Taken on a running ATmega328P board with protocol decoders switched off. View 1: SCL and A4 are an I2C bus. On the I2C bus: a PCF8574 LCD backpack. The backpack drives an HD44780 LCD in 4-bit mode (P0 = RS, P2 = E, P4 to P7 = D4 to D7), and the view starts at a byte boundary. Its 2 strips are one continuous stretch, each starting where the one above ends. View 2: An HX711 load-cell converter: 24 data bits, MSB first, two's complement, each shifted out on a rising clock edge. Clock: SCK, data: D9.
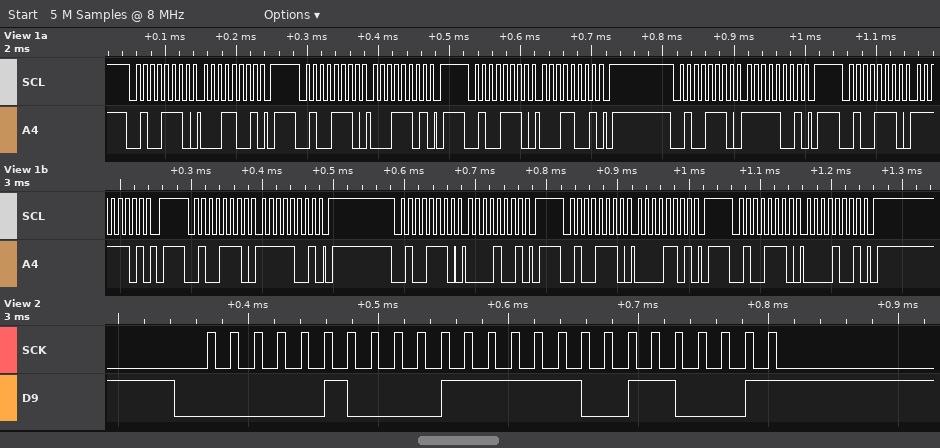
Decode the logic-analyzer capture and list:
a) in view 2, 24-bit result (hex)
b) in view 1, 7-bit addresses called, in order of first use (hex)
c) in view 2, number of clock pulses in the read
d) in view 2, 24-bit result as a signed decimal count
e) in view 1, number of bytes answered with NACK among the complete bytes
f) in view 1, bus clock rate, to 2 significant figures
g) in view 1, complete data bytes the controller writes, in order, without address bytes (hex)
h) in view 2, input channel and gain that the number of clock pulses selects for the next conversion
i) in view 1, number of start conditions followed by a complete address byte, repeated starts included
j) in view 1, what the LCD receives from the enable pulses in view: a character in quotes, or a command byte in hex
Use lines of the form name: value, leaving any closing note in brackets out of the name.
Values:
in view 2, 24-bit result: 0x043F31
in view 1, 7-bit addresses called, in order of first use: 0x27
in view 2, number of clock pulses in the read: 25
in view 2, 24-bit result as a signed decimal count: 278321
in view 1, number of bytes answered with NACK among the complete bytes: 0
in view 1, bus clock rate, to 2 significant figures: 100 kHz
in view 1, complete data bytes the controller writes, in order, without address bytes: 19 1D 19 F9 FD F9 09 0D 09
in view 2, input channel and gain that the number of clock pulses selects for the next conversion: channel A, gain 128
in view 1, number of start conditions followed by a complete address byte, repeated starts included: 9
in view 1, what the LCD receives from the enable pulses in view: a character in quotes, or a command byte in hex: data 0x1F
